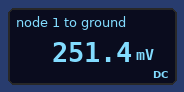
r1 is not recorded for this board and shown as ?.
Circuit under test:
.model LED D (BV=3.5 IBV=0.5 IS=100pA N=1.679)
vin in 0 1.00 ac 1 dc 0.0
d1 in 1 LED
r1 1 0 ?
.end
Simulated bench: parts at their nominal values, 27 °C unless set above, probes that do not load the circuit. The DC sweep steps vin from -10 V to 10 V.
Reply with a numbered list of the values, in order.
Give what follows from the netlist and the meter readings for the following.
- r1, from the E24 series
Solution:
1. 82 Ω
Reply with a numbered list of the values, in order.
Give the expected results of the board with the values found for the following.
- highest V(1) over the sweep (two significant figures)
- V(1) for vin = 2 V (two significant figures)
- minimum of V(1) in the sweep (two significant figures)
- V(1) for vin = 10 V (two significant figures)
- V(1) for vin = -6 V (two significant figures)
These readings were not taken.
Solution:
1. 9.1 V
2. 1.2 V
3. -6.6 V
4. 9.1 V
5. -2.6 V
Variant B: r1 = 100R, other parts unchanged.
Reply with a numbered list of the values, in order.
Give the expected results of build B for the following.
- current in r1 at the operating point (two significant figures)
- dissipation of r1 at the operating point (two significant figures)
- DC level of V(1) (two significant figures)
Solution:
1. 2.6 mA
2. 670 µW
3. 260 mV
